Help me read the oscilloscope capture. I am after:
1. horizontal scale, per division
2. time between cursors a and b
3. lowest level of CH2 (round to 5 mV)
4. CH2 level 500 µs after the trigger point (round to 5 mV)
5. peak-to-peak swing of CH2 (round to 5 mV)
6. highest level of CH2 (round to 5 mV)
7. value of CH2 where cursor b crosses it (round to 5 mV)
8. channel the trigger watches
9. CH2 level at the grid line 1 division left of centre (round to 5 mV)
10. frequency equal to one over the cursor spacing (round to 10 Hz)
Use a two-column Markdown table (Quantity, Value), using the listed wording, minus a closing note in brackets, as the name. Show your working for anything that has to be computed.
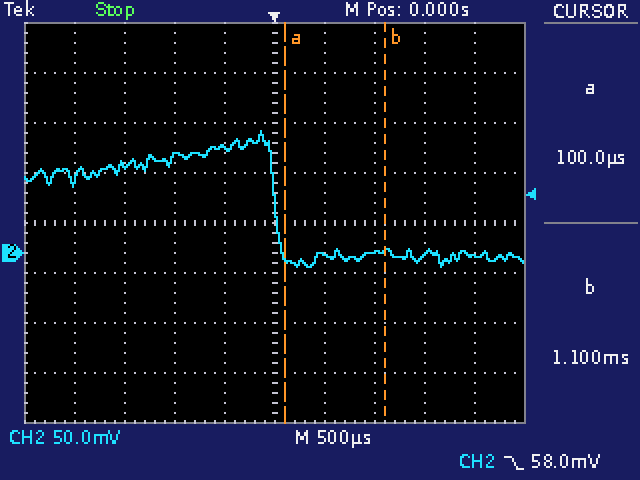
| Quantity | Value |
|---|---|
| horizontal scale, per division | 500 µs |
| time between cursors a and b | 1.1 ms − (100 µs) = 1.00 ms |
| lowest level of CH2 | -15 mV |
| CH2 level 500 µs after the trigger point | 0 mV |
| peak-to-peak swing of CH2 | 120 mV − (-15 mV) = 135 mV |
| highest level of CH2 | 120 mV |
| value of CH2 where cursor b crosses it | 0 mV |
| channel the trigger watches | CH2 |
| CH2 level at the grid line 1 division left of centre | 105 mV |
| frequency equal to one over the cursor spacing | 1 / 1.00 ms ≈ 1.00 kHz |
